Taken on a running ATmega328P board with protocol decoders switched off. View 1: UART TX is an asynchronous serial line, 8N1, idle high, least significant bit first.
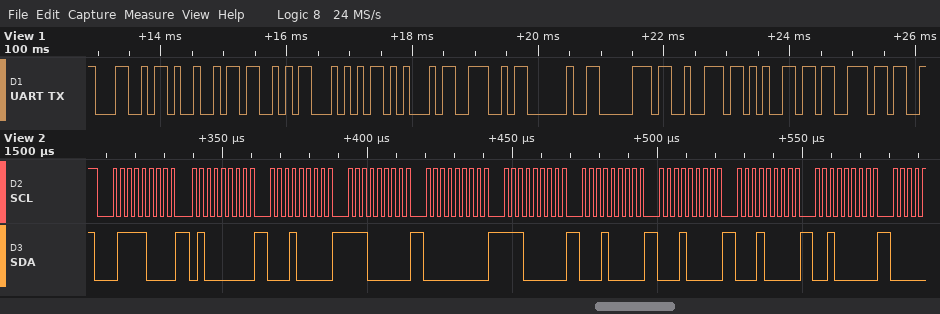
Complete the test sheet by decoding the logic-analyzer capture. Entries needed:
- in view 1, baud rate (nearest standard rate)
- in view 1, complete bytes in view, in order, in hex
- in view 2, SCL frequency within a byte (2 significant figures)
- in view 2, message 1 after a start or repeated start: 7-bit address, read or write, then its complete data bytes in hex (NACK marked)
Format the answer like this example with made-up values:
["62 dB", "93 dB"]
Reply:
["9600 baud", "0x4C 0x49 0x53 0x54 0x45 0x4E 0x20 0x70 0x72 0x65 0x73", "400 kHz", "0x3C write: 40 10 E0 00 E0 10 10 10 20"]
